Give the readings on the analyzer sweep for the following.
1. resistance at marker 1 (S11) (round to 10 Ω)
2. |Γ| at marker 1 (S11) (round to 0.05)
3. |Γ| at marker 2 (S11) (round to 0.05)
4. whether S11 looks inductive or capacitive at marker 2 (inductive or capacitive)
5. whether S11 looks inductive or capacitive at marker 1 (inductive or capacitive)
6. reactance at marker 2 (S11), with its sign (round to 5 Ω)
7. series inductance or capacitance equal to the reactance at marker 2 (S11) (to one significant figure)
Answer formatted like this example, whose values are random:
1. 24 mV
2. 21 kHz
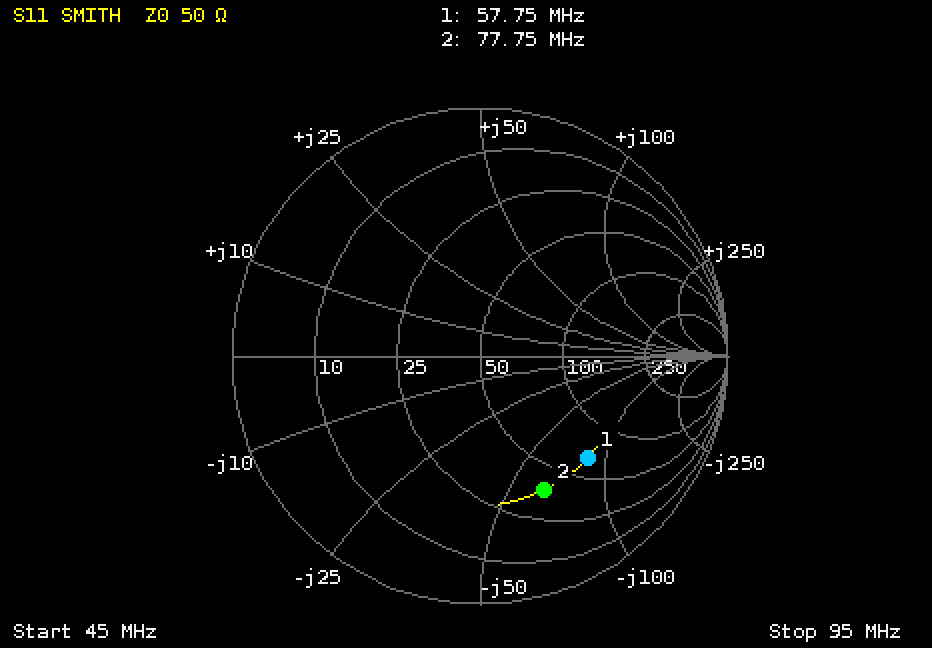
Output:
1. 70 Ω
2. 0.60
3. 0.60
4. capacitive
5. capacitive
6. -65 Ω
7. 30 pF
